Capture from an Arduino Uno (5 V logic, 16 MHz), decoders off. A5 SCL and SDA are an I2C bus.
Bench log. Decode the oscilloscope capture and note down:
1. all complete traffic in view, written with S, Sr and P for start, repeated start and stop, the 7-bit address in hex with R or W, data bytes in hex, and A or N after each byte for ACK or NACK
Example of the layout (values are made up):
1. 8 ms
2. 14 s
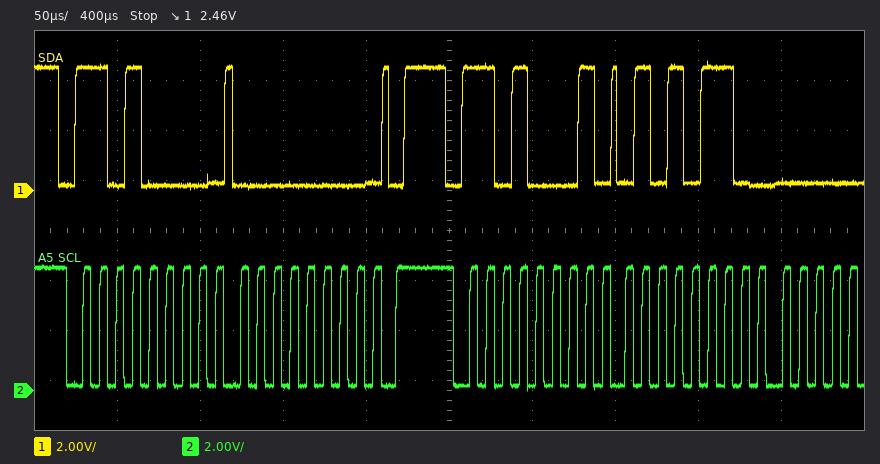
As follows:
1. S 68W A 00 A P S 68R A 56 A
